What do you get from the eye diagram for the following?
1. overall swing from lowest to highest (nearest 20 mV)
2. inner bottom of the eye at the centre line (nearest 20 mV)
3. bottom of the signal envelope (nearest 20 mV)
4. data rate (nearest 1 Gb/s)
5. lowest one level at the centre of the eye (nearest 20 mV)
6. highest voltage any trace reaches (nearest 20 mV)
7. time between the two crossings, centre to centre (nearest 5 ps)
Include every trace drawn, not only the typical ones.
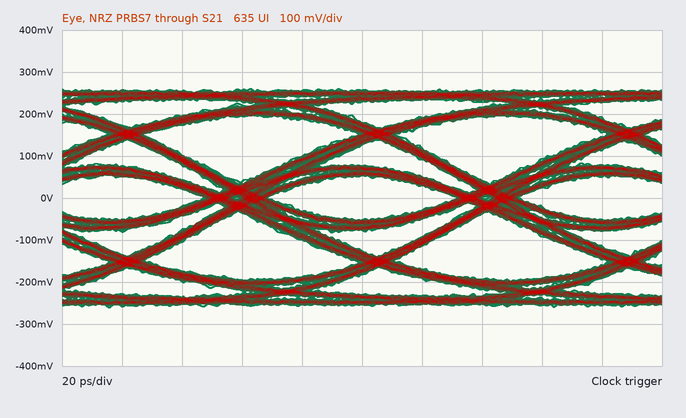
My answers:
520 mV
-60 mV
-260 mV
12 Gb/s
60 mV
260 mV
85 ps
